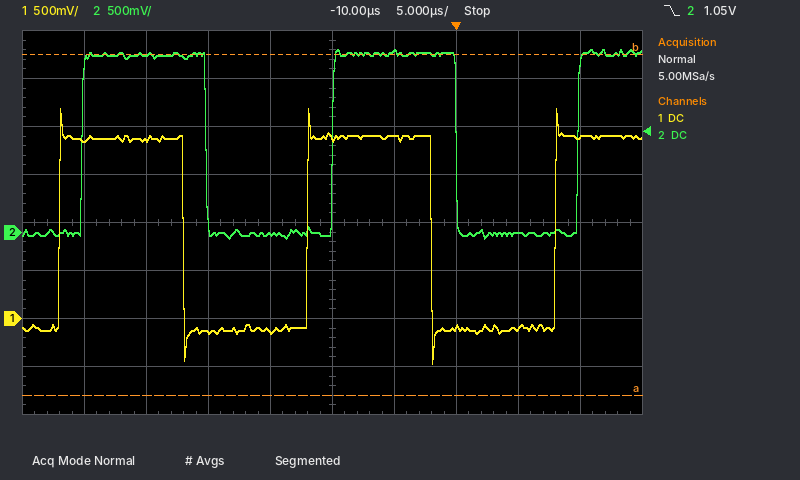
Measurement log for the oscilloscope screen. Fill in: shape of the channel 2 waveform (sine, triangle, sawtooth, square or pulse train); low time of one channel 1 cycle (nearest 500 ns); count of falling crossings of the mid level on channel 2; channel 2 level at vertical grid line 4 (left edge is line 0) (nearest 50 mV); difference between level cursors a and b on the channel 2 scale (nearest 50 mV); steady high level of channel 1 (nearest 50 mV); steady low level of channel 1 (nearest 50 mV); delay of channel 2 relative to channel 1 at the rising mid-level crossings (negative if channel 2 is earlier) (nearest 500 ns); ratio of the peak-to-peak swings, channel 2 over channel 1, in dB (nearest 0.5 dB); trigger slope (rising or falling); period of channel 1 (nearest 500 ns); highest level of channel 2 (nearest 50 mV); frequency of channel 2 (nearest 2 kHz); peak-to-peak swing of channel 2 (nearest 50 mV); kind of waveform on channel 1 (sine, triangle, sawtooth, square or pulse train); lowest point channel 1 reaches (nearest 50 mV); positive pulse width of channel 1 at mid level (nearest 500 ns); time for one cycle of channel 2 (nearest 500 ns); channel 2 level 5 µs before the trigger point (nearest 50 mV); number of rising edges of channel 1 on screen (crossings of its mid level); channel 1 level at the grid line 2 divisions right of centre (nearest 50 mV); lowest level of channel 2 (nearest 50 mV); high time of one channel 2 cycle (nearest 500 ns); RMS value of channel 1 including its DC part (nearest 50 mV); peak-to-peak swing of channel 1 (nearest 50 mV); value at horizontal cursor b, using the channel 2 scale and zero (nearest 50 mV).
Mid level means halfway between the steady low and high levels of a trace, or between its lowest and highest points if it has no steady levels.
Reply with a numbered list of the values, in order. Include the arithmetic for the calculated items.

1. square
2. 10.0 µs
3. 2
4. 0 mV
5. 3.55 V
6. 1.90 V
7. -100 mV
8. +2.0 µs
9. 20 log10(1.95 V / 2.65 V) ≈ -2.66 dB, so -2.5 dB to the nearest 0.5 dB
10. falling
11. 20.0 µs
12. 1.90 V
13. 1 / 20.0 µs ≈ 50 kHz
14. 1.90 V − (-50 mV) = 1.95 V
15. square
16. -450 mV
17. 10.0 µs
18. 20.0 µs
19. 1.90 V
20. 3
21. -100 mV
22. -50 mV
23. 10.0 µs
24. √(0.5 × (1.90 V)² + 0.5 × (-100 mV)²) ≈ 1.35 V
25. 2.20 V − (-450 mV) = 2.65 V
26. 1.85 V
